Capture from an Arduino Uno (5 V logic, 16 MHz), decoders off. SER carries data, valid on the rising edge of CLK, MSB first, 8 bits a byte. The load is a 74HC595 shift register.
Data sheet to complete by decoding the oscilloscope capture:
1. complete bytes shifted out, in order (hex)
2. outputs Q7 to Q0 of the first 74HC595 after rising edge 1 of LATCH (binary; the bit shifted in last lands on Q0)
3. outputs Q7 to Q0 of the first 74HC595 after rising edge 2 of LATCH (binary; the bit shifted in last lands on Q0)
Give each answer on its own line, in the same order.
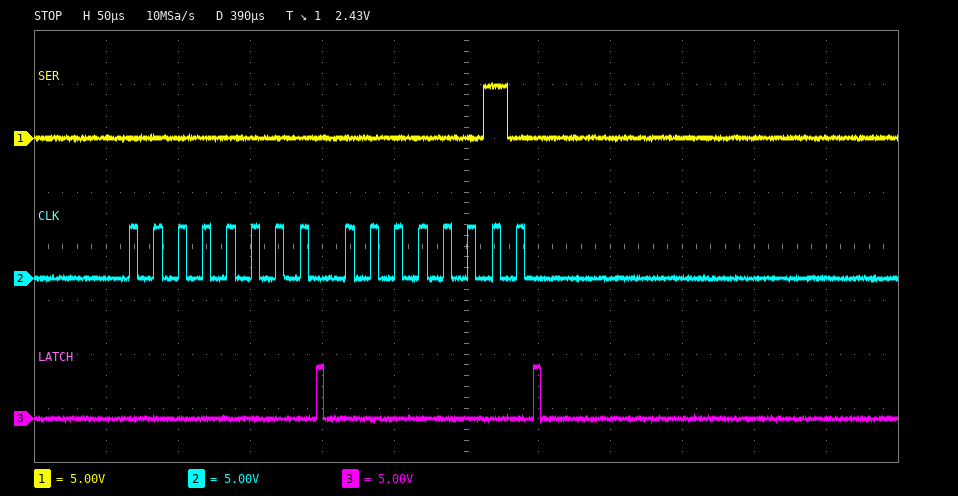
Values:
00 02
00000000
00000010
